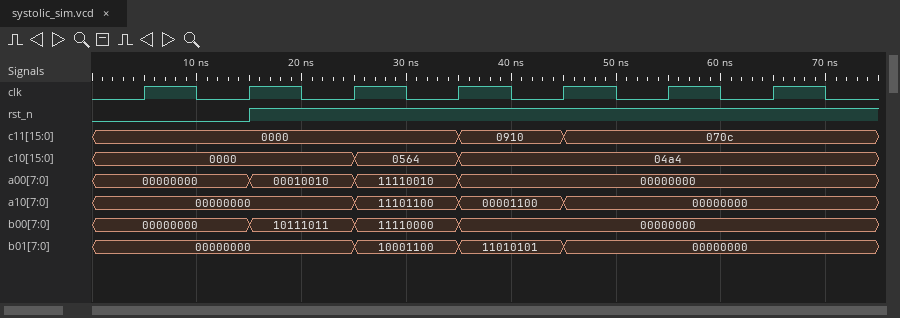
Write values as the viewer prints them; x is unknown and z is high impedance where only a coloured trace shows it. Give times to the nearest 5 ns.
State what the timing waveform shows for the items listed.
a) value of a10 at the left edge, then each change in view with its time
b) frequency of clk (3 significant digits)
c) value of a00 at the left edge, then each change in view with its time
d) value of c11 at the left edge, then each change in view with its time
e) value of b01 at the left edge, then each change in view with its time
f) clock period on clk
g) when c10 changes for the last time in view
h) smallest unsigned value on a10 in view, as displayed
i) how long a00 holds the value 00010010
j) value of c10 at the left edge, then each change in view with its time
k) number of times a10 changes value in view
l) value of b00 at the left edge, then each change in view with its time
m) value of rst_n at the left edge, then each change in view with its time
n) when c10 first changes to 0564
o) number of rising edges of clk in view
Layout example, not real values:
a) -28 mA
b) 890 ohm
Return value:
a) 00000000, 11101100 at 25 ns, 00001100 at 35 ns, 00000000 at 45 ns
b) 100 MHz
c) 00000000, 00010010 at 15 ns, 11110010 at 25 ns, 00000000 at 35 ns
d) 0000, 0910 at 35 ns, 070c at 45 ns
e) 00000000, 10001100 at 25 ns, 11010101 at 35 ns, 00000000 at 45 ns
f) 10 ns
g) 35 ns
h) 00000000
i) 10 ns
j) 0000, 0564 at 25 ns, 04a4 at 35 ns
k) 3
l) 00000000, 10111011 at 15 ns, 11110000 at 25 ns, 00000000 at 35 ns
m) 0, 1 at 15 ns
n) 25 ns
o) 7
